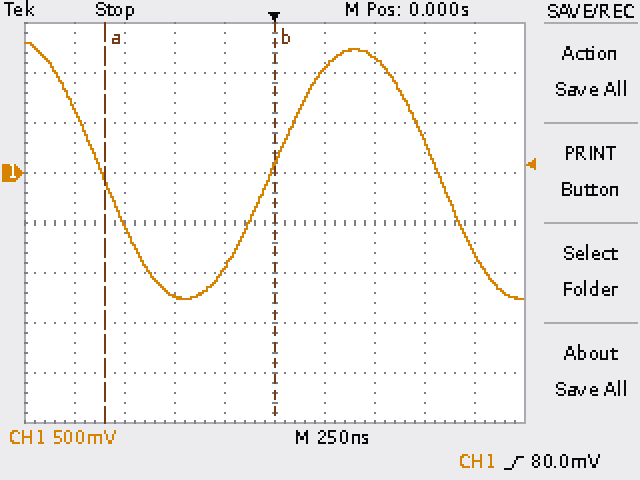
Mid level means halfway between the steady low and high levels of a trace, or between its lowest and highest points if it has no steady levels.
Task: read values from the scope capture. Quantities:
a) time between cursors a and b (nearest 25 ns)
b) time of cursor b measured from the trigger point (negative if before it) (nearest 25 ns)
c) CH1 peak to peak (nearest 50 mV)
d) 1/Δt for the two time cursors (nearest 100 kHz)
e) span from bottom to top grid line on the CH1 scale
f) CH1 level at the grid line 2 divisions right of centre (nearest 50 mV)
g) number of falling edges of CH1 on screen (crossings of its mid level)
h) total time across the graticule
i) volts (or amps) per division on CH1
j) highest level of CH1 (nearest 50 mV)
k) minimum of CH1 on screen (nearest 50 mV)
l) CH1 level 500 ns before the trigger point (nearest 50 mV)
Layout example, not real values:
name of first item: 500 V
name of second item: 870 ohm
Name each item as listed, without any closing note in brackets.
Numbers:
time between cursors a and b: 850 ns
time of cursor b measured from the trigger point (negative if before it): 0 ns
CH1 peak to peak: 2.55 V
1/Δt for the two time cursors: 1.2 MHz
span from bottom to top grid line on the CH1 scale: 4 V
CH1 level at the grid line 2 divisions right of centre: 1.15 V
number of falling edges of CH1 on screen: 2
total time across the graticule: 2.5 µs
volts (or amps) per division on CH1: 500 mV
highest level of CH1: 1.30 V
minimum of CH1 on screen: -1.25 V
CH1 level 500 ns before the trigger point: -1.25 V
